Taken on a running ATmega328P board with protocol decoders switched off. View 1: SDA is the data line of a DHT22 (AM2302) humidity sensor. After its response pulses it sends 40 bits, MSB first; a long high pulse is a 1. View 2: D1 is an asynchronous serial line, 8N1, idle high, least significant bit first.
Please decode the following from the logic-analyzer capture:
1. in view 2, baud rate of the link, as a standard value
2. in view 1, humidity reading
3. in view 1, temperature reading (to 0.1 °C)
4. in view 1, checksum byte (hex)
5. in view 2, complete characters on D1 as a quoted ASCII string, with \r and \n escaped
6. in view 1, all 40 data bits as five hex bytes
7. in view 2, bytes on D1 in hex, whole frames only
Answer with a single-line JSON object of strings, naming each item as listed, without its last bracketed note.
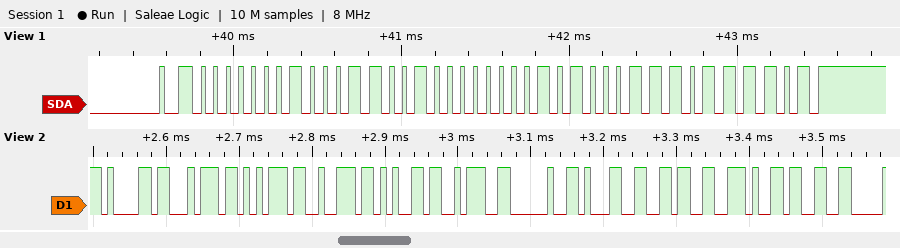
{"in view 2, baud rate of the link, as a standard value": "115200 baud", "in view 1, humidity reading": "28.1 %", "in view 1, temperature reading": "16.3 °C", "in view 1, checksum byte": "0xBD", "in view 2, complete characters on D1 as a quoted ASCII string, with \\r and \\n escaped": "\"ature: 16.3\"", "in view 1, all 40 data bits as five hex bytes": "01 19 00 A3 BD", "in view 2, bytes on D1 in hex, whole frames only": "0x61 0x74 0x75 0x72 0x65 0x3A 0x20 0x31 0x36 0x2E 0x33"}
